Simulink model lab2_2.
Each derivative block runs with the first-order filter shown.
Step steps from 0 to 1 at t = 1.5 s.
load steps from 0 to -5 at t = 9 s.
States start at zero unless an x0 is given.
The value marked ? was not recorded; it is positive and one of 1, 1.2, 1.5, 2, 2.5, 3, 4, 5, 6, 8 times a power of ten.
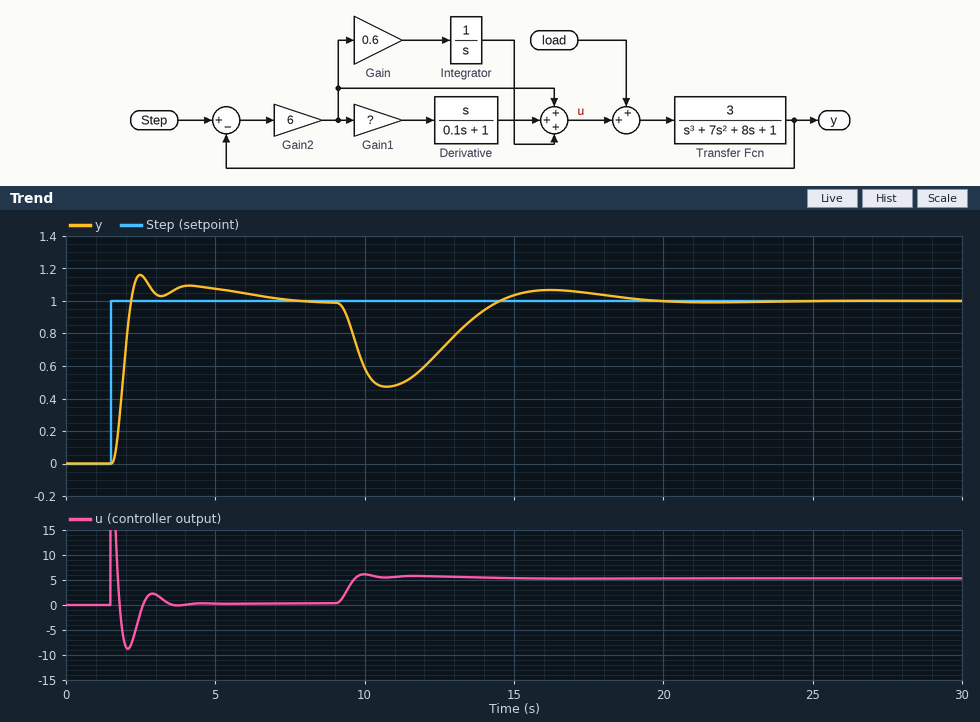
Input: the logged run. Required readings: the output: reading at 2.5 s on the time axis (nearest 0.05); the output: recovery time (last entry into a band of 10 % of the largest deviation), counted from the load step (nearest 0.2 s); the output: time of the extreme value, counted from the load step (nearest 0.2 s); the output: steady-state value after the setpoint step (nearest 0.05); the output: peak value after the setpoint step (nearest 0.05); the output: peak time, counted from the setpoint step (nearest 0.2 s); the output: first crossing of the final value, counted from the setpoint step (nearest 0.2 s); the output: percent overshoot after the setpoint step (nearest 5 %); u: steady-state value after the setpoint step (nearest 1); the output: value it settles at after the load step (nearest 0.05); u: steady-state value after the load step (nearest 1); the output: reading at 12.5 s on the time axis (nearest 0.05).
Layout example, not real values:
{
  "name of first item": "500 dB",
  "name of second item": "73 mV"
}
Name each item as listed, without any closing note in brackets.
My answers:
{
  "the output: reading at 2.5 s on the time axis": "1.15",
  "the output: recovery time (last entry into a band of 10 % of the largest deviation), counted from the load step": "8.4 s",
  "the output: time of the extreme value, counted from the load step": "1.8 s",
  "the output: steady-state value after the setpoint step": "1.00",
  "the output: peak value after the setpoint step": "1.15",
  "the output: peak time, counted from the setpoint step": "1.0 s",
  "the output: first crossing of the final value, counted from the setpoint step": "0.6 s",
  "the output: percent overshoot after the setpoint step": "15 %",
  "u: steady-state value after the setpoint step": "0",
  "the output: value it settles at after the load step": "1.00",
  "u: steady-state value after the load step": "5",
  "the output: reading at 12.5 s on the time axis": "0.70"
}
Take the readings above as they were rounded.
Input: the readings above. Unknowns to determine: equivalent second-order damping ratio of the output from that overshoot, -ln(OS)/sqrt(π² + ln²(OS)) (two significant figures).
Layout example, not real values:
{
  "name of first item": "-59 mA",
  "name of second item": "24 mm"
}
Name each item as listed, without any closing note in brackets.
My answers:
{
  "equivalent second-order damping ratio of the output from that overshoot, -ln(OS)/sqrt(π² + ln²(OS))": "0.52"
}
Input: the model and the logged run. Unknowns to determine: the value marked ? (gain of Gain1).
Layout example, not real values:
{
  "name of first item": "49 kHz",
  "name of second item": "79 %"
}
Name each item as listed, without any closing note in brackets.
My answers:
{
  "the value marked ?": "1"
}
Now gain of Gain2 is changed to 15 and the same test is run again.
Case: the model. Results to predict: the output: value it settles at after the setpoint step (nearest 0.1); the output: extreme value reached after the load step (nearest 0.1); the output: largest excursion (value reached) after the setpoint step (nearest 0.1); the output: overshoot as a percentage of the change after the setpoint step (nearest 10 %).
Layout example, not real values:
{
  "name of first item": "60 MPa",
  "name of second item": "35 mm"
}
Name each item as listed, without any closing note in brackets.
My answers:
{
  "the output: value it settles at after the setpoint step": "1.0",
  "the output: extreme value reached after the load step": "0.8",
  "the output: largest excursion (value reached) after the setpoint step": "1.5",
  "the output: overshoot as a percentage of the change after the setpoint step": "50 %"
}
